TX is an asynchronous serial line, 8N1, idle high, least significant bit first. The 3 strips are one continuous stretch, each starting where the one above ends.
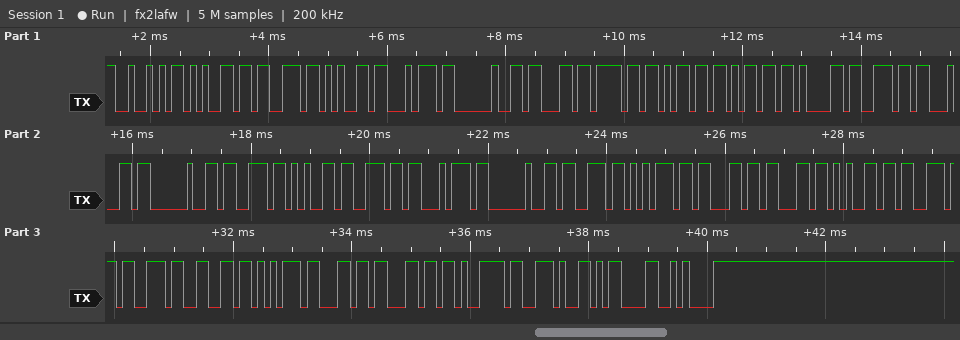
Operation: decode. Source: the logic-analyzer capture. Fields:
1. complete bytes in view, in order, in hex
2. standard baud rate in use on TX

52 65 73 65 74 20 63 6F 6D 6D 61 6E 64 20 73 65 6E 74 20 73 75 63 63 65 73 73 66 75 6C 6C 79 2E 0D 0A
9600 baud
